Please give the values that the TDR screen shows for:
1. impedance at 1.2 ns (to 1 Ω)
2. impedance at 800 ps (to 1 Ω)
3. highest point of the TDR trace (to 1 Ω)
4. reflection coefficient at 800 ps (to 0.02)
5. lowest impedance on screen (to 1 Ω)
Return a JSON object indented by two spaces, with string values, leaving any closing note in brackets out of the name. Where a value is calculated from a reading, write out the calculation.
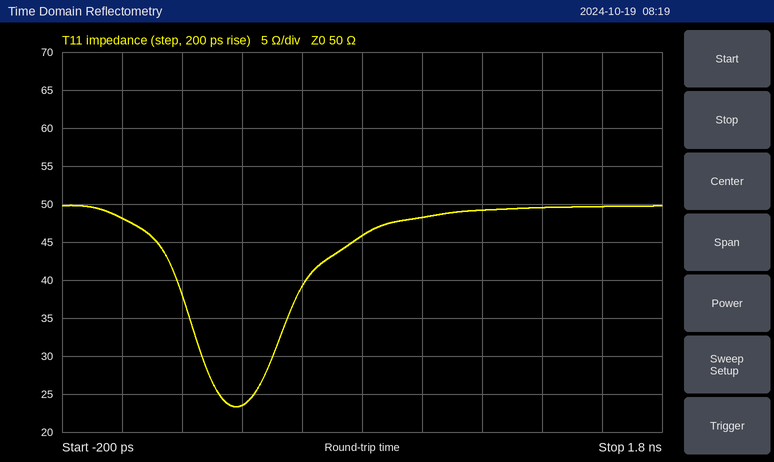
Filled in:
{
  "impedance at 1.2 ns": "49 Ω",
  "impedance at 800 ps": "46 Ω",
  "highest point of the TDR trace": "50 Ω",
  "reflection coefficient at 800 ps": "(46 − 50)/(46 + 50) ≈ -0.04",
  "lowest impedance on screen": "23 Ω"
}
